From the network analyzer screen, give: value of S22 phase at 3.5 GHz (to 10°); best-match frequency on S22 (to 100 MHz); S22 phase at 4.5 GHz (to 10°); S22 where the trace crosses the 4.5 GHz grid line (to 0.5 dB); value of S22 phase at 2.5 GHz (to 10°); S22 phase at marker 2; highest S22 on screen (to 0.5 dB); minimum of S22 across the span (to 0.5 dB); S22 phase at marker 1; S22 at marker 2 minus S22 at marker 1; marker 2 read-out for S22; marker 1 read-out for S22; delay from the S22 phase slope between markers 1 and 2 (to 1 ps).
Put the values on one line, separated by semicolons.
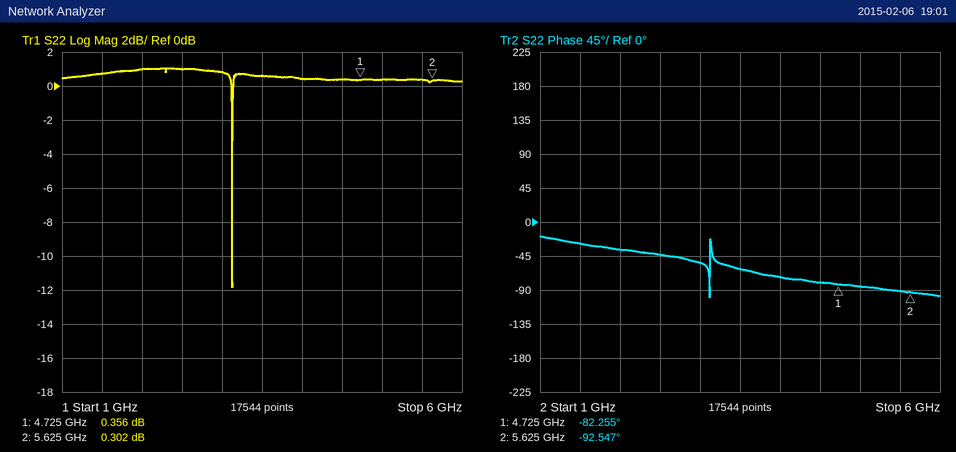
-60°; 3.1 GHz; -80°; 0.5 dB; -40°; -92.547°; 1.0 dB; -12.0 dB; -82.255°; -0.054 dB; 0.302 dB; 0.356 dB; 32 ps
